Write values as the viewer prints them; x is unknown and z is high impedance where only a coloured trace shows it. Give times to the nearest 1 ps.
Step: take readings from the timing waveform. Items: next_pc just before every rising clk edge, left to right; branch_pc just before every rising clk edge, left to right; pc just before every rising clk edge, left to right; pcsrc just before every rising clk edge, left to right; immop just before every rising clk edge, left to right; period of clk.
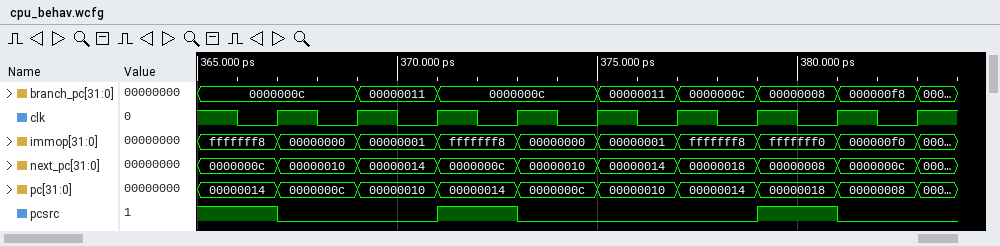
0000000c, 00000010, 00000014, 0000000c, 00000010, 00000014, 00000018, 00000008, 0000000c
0000000c, 0000000c, 00000011, 0000000c, 0000000c, 00000011, 0000000c, 00000008, 000000f8
00000014, 0000000c, 00000010, 00000014, 0000000c, 00000010, 00000014, 00000018, 00000008
1 0 0 1 0 0 0 1 0
fffffff8, 00000000, 00000001, fffffff8, 00000000, 00000001, fffffff8, fffffff0, 000000f0
2 ps
